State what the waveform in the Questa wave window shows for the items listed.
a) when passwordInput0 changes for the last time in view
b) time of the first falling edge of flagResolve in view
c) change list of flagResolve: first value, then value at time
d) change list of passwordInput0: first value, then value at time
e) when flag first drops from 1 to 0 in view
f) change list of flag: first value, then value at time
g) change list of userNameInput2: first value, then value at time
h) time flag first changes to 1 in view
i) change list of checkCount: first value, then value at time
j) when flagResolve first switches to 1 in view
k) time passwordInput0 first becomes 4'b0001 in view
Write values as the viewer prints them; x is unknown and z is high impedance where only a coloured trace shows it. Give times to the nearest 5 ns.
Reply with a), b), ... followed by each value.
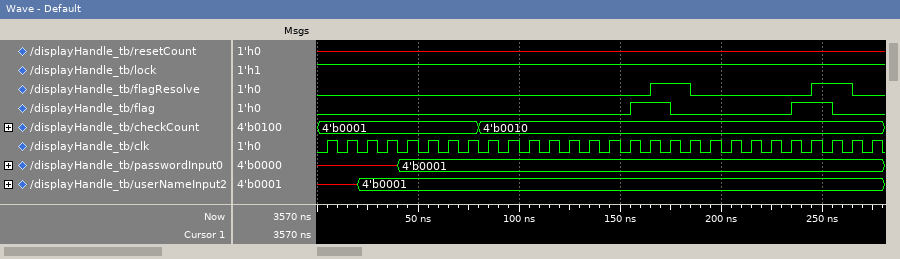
a) 40 ns
b) 185 ns
c) 0, 1 at 165 ns, 0 at 185 ns, 1 at 245 ns, 0 at 265 ns
d) x, 4'b0001 at 40 ns
e) 175 ns
f) 0, 1 at 155 ns, 0 at 175 ns, 1 at 235 ns, 0 at 255 ns
g) x, 4'b0001 at 20 ns
h) 155 ns
i) 4'b0001, 4'b0010 at 80 ns
j) 165 ns
k) 40 ns
